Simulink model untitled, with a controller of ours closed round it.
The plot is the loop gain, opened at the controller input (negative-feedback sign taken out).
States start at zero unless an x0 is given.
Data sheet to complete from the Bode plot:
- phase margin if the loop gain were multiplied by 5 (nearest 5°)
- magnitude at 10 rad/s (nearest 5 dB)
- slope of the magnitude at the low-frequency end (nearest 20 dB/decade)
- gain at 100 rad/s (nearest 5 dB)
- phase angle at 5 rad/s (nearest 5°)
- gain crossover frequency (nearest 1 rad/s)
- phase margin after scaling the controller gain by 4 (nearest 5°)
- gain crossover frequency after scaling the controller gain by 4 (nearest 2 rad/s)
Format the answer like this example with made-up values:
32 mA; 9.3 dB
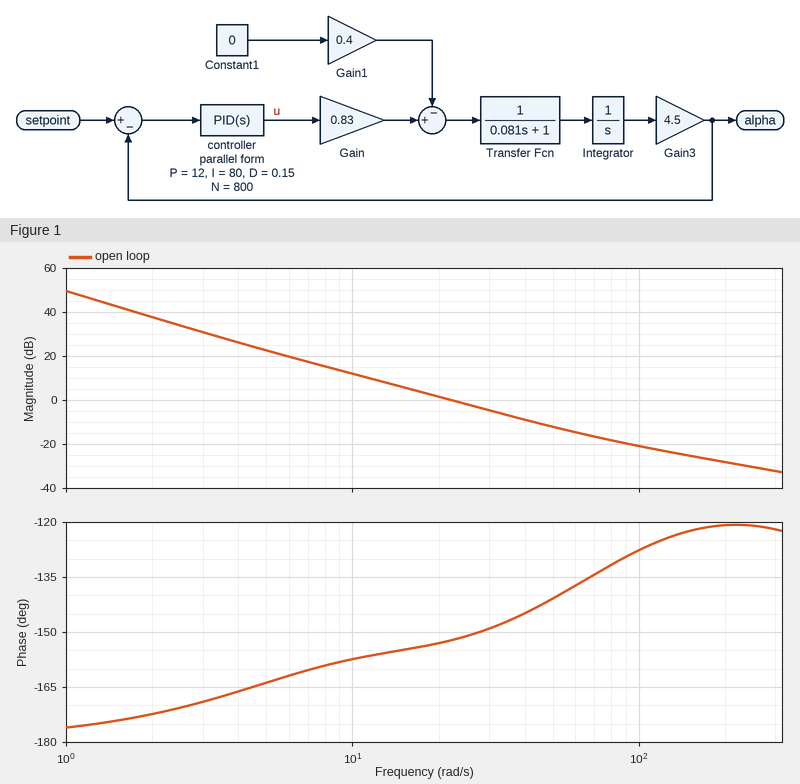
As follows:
40°; 10 dB; -40 dB/decade; -20 dB; -165°; 22 rad/s; 40°; 50 rad/s
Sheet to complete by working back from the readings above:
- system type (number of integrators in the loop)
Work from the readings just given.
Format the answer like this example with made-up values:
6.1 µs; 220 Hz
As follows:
2
